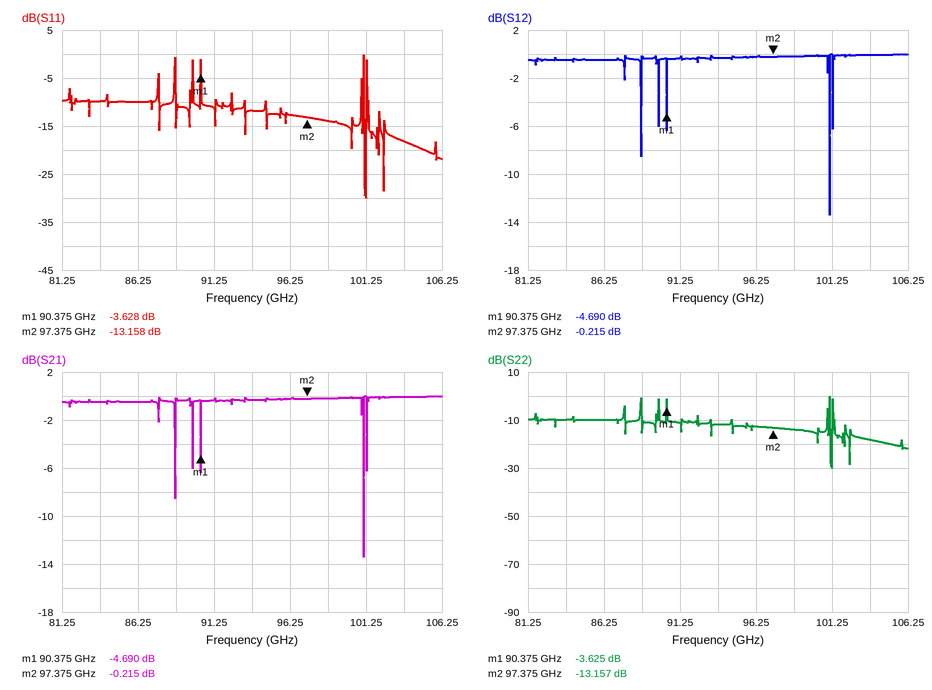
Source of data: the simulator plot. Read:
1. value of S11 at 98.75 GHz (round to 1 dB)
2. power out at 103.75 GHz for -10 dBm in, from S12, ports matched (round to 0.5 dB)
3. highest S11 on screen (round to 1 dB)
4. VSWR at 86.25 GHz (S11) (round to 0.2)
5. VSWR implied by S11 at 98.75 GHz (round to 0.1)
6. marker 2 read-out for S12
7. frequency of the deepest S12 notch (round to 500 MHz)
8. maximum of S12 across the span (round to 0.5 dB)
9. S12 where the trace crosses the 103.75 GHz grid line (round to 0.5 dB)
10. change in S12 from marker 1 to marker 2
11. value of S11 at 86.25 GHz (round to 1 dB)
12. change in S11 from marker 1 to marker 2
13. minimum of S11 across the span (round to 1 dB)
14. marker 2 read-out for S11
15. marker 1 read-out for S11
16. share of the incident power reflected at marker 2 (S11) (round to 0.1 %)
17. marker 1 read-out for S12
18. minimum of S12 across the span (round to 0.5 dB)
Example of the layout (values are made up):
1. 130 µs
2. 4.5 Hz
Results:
1. -14 dB
2. -10.0 dBm
3. 0 dB
4. 2.0
5. 1.5
6. -0.215 dB
7. 101.0 GHz
8. 0.0 dB
9. 0.0 dB
10. 4.475 dB
11. -10 dB
12. -9.530 dB
13. -30 dB
14. -13.158 dB
15. -3.628 dB
16. 4.8 %
17. -4.690 dB
18. -13.5 dB
